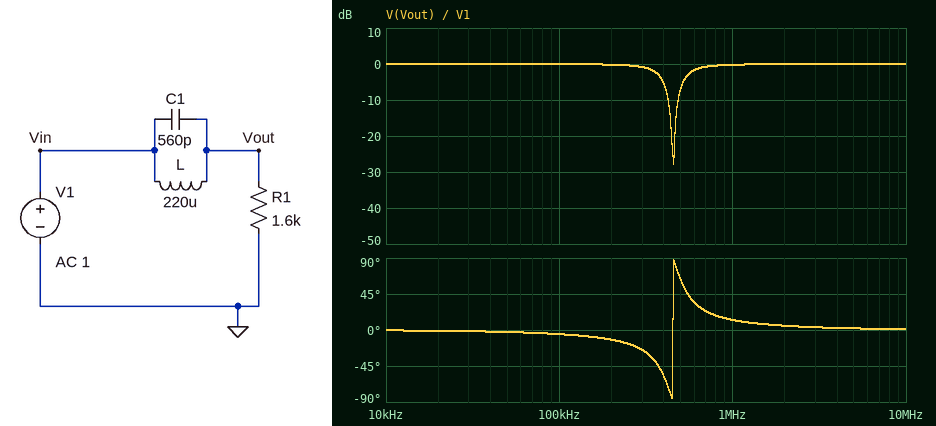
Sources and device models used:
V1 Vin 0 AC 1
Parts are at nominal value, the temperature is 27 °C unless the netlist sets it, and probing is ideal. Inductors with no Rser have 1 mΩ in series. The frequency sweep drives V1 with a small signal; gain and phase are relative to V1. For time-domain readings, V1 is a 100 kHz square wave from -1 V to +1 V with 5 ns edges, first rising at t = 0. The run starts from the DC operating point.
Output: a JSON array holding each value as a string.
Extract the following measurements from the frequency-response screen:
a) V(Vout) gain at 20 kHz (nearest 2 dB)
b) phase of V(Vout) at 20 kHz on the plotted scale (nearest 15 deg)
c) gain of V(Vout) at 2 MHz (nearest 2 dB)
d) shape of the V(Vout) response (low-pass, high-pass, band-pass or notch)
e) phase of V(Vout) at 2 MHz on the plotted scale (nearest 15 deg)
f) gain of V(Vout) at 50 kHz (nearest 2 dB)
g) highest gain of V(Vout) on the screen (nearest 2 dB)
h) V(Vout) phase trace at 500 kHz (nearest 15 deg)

["0 dB", "0 deg", "0 dB", "notch", "0 deg", "0 dB", "0 dB", "60 deg"]
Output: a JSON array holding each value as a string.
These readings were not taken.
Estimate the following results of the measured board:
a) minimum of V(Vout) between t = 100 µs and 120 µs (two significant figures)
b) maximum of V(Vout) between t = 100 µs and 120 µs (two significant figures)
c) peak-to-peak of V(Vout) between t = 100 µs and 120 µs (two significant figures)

["-1.3 V", "1.3 V", "2.6 V"]
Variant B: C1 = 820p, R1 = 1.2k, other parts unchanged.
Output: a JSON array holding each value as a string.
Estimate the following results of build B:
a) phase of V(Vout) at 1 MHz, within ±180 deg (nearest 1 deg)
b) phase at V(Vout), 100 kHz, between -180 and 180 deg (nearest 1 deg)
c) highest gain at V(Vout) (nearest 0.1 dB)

["11 deg", "-7 deg", "0 dB"]
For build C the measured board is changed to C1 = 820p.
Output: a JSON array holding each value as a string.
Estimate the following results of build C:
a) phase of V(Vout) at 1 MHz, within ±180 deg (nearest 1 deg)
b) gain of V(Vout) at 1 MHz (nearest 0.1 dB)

["8 deg", "-0.1 dB"]
